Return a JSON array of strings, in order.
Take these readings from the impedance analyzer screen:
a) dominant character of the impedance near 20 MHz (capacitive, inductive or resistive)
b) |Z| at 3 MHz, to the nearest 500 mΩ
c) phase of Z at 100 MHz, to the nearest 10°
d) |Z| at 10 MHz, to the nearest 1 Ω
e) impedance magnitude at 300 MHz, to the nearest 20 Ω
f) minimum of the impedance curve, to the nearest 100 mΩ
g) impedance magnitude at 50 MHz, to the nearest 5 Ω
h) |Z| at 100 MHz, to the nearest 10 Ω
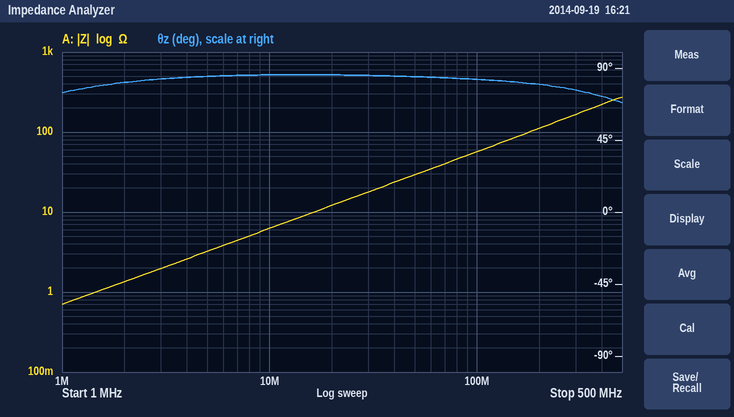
["inductive", "2.0 Ω", "80°", "6 Ω", "160 Ω", "700 mΩ", "30 Ω", "60 Ω"]
